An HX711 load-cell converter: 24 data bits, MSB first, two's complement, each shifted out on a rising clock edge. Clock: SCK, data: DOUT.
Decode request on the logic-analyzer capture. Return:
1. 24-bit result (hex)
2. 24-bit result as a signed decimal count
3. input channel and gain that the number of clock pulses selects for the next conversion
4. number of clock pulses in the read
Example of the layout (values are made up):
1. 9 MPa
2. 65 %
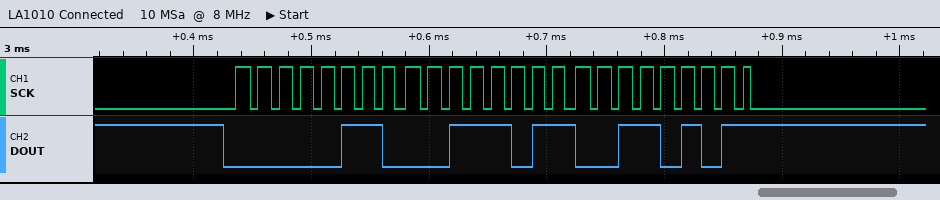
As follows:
1. 0x063B35
2. 408373
3. channel A, gain 128
4. 25
